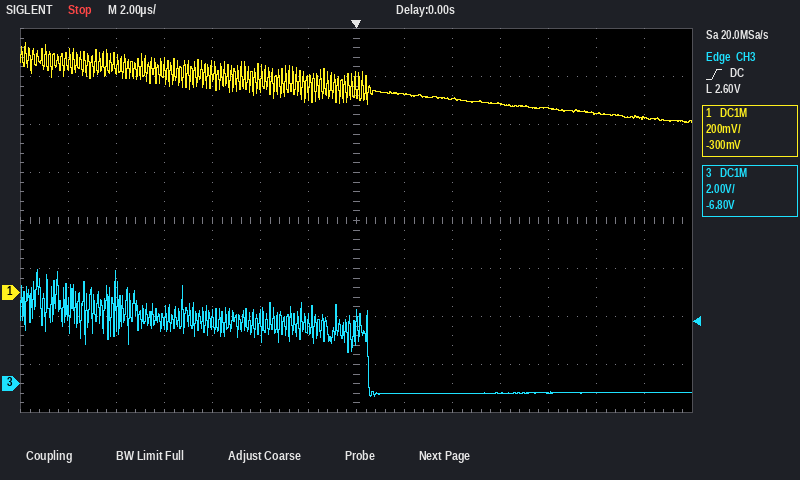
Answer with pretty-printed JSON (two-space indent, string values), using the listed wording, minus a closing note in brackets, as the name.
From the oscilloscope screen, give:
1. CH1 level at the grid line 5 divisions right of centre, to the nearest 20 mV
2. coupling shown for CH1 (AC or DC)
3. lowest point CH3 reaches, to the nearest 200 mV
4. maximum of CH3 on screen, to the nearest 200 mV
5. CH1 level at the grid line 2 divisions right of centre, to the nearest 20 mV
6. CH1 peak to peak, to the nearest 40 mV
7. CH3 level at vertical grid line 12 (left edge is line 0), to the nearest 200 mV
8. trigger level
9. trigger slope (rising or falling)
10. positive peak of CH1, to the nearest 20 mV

{
  "CH1 level at the grid line 5 divisions right of centre, to the nearest 20 mV": "740 mV",
  "coupling shown for CH1": "DC",
  "lowest point CH3 reaches, to the nearest 200 mV": "-600 mV",
  "maximum of CH3 on screen, to the nearest 200 mV": "4.8 V",
  "CH1 level at the grid line 2 divisions right of centre, to the nearest 20 mV": "800 mV",
  "CH1 peak to peak, to the nearest 40 mV": "320 mV",
  "CH3 level at vertical grid line 12 (left edge is line 0), to the nearest 200 mV": "-400 mV",
  "trigger level": "2.60 V",
  "trigger slope": "rising",
  "positive peak of CH1, to the nearest 20 mV": "1.04 V"
}
